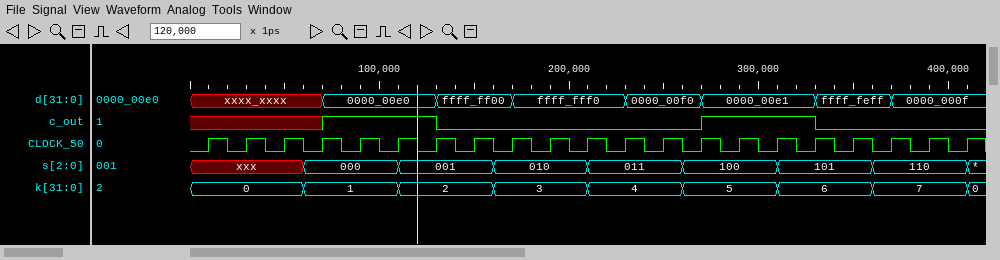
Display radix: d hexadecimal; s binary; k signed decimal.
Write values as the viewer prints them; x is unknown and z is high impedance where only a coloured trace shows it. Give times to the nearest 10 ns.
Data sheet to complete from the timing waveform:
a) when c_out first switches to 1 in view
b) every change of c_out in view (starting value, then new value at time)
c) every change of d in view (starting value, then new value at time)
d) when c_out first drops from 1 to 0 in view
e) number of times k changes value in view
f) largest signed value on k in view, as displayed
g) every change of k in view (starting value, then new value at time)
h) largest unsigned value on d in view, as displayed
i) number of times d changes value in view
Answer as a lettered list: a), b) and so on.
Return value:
a) 70 ns
b) x, 1 at 70 ns, 0 at 130 ns, 1 at 270 ns, 0 at 330 ns
c) xxxx_xxxx, 0000_00e0 at 70 ns, ffff_ff00 at 130 ns, ffff_fff0 at 170 ns, 0000_00f0 at 230 ns, 0000_00e1 at 270 ns, ffff_feff at 330 ns, 0000_000f at 370 ns
d) 130 ns
e) 8
f) 7
g) 0, 1 at 60 ns, 2 at 110 ns, 3 at 160 ns, 4 at 210 ns, 5 at 260 ns, 6 at 310 ns, 7 at 360 ns, 0 at 410 ns
h) ffff_fff0
i) 7
